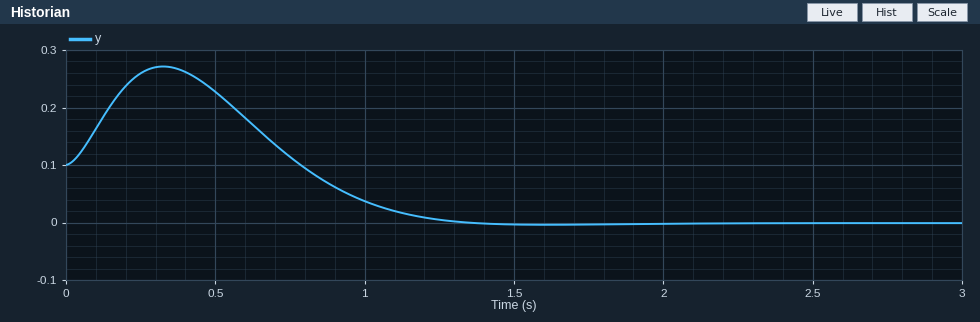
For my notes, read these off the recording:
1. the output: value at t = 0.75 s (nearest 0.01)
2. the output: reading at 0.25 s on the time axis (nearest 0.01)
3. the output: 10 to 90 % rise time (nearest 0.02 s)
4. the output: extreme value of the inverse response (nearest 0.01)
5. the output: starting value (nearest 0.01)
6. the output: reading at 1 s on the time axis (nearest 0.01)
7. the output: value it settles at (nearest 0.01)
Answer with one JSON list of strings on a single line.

["0.11", "0.26", "0.38 s", "0.27", "0.10", "0.04", "0.00"]
